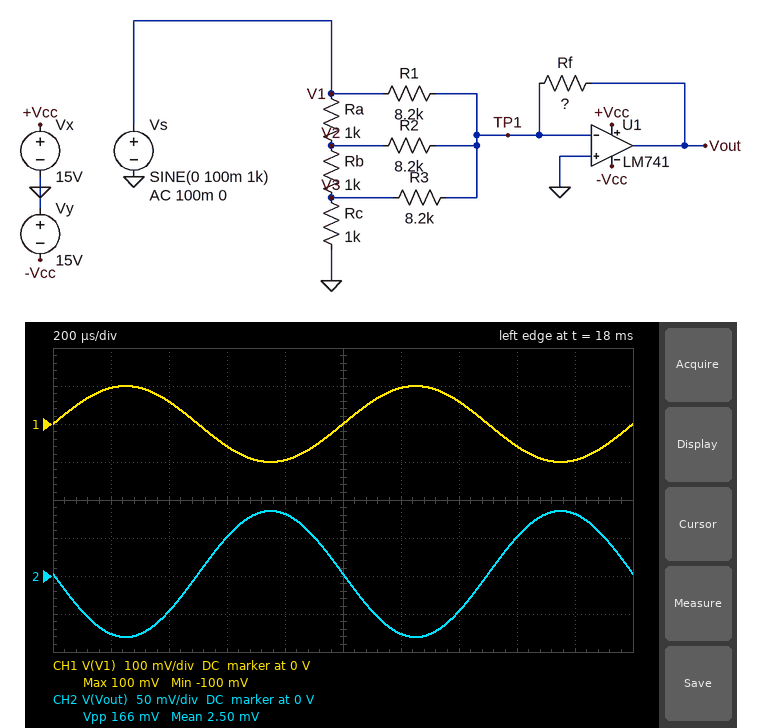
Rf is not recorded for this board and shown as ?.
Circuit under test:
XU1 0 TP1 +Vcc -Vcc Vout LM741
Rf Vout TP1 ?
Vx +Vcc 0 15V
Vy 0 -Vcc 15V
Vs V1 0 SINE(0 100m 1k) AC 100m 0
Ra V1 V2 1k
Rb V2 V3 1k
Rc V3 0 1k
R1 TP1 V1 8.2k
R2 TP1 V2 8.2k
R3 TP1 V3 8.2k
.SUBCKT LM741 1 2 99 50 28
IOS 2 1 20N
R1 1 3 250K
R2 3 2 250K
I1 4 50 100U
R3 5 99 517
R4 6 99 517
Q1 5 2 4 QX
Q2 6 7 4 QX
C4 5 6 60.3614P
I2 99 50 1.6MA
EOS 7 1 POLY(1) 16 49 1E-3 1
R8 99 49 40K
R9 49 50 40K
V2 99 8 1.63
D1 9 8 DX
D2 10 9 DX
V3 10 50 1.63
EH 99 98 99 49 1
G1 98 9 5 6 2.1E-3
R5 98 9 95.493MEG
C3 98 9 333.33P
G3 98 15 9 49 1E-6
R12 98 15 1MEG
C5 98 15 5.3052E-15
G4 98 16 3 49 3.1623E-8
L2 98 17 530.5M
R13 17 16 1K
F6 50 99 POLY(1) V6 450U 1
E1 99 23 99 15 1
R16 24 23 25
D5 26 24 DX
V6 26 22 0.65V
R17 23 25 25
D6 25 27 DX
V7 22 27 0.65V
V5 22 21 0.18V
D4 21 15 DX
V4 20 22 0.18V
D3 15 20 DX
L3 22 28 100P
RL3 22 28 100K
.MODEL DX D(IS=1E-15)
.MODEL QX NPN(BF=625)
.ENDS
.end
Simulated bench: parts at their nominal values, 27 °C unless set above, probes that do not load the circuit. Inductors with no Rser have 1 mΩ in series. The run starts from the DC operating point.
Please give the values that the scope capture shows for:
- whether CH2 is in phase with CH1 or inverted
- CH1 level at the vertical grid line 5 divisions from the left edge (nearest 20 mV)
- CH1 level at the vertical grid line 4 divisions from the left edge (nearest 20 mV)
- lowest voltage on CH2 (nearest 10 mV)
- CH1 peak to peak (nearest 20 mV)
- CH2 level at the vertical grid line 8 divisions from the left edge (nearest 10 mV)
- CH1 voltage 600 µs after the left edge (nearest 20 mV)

inverted
0 V
-100 mV
-80 mV
200 mV
50 mV
-60 mV
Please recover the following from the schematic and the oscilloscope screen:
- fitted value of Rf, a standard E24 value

3.6 kΩ
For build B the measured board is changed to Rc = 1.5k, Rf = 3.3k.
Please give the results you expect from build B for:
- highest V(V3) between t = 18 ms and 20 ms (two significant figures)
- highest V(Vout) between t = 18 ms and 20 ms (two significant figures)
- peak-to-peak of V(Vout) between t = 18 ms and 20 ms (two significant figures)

36 mV
83 mV
160 mV
